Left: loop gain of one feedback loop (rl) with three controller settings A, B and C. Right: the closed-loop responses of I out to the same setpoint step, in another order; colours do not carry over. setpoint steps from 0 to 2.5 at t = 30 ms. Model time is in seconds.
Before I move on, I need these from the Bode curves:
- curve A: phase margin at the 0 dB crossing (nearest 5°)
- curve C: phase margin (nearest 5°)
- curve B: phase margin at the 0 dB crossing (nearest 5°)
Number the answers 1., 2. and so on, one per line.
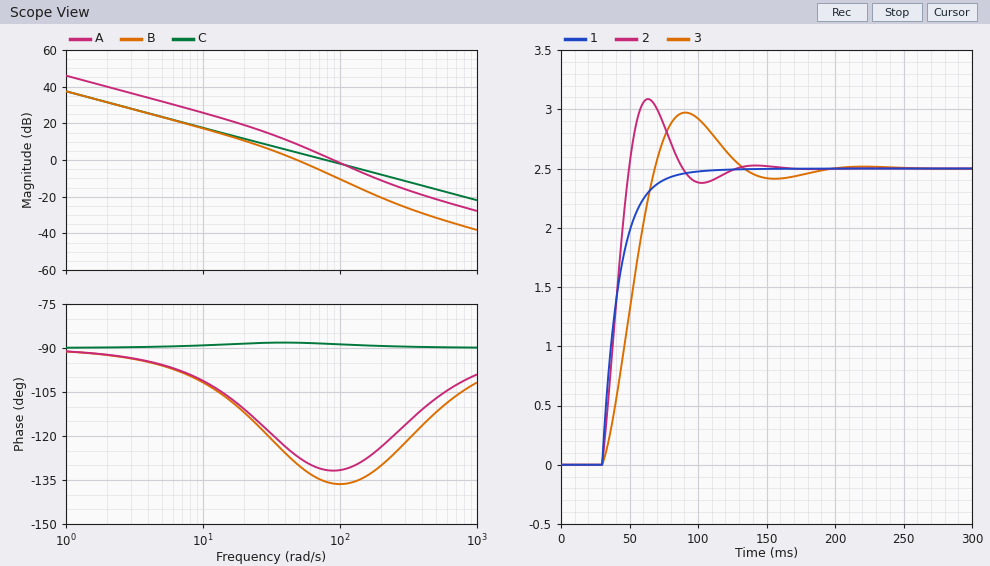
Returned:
1. 50°
2. 90°
3. 50°
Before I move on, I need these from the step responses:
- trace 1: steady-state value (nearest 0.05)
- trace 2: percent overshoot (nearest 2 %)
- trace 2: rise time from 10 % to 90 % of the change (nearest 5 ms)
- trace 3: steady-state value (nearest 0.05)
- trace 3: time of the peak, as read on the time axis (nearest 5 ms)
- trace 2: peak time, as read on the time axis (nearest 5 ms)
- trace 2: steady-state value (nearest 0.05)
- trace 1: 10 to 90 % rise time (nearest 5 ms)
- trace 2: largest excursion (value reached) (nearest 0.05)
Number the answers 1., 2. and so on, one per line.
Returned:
1. 2.50
2. 24 %
3. 15 ms
4. 2.50
5. 90 ms
6. 65 ms
7. 2.50
8. 30 ms
9. 3.10
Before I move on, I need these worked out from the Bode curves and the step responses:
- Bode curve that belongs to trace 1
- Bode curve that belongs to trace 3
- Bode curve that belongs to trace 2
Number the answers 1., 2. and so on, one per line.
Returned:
1. C
2. B
3. A
